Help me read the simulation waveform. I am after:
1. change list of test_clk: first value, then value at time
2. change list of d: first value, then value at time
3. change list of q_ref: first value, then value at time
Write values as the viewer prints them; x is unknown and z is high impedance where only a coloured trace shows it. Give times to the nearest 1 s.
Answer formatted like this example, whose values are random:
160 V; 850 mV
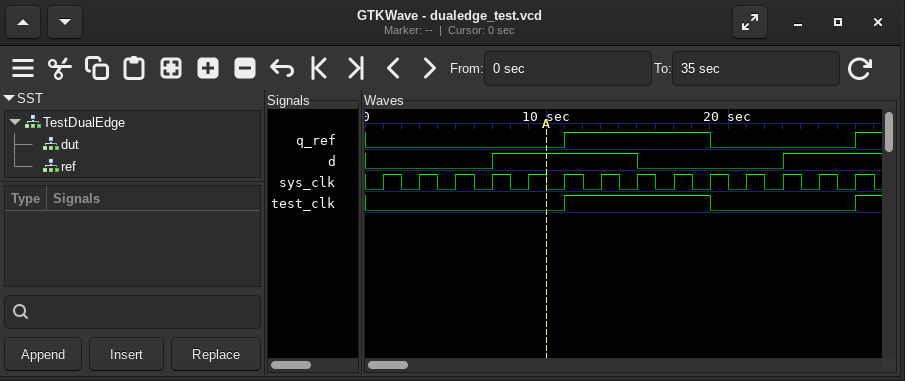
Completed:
0, 1 at 11 s, 0 at 19 s, 1 at 27 s; 0, 1 at 7 s, 0 at 15 s, 1 at 23 s; 0, 1 at 11 s, 0 at 19 s, 1 at 27 s
